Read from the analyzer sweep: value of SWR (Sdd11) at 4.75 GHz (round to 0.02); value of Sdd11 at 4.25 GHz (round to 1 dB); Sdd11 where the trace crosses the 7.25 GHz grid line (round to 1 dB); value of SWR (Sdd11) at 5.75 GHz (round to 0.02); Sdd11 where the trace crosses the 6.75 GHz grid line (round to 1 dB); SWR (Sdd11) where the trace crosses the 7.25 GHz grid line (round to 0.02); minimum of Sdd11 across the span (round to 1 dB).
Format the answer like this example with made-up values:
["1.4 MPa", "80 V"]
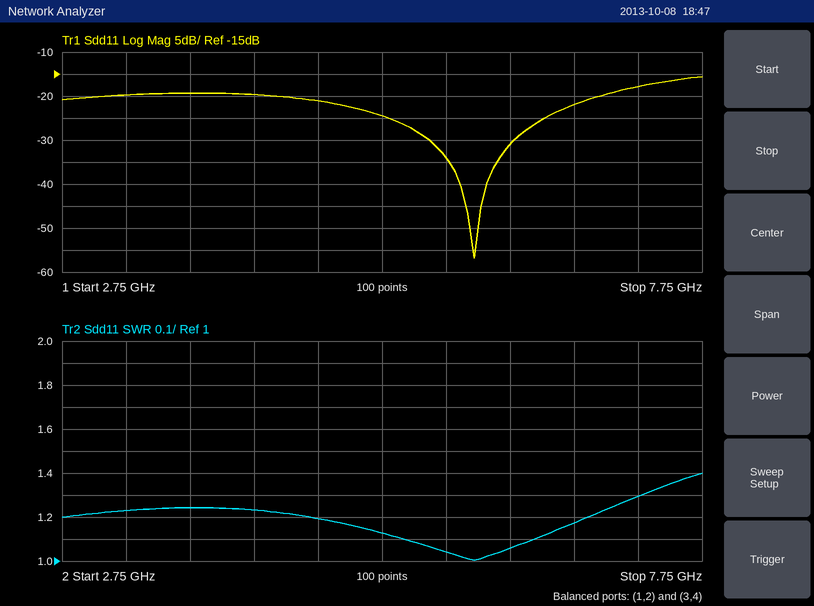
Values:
["1.20", "-20 dB", "-18 dB", "1.04", "-22 dB", "1.30", "-57 dB"]
